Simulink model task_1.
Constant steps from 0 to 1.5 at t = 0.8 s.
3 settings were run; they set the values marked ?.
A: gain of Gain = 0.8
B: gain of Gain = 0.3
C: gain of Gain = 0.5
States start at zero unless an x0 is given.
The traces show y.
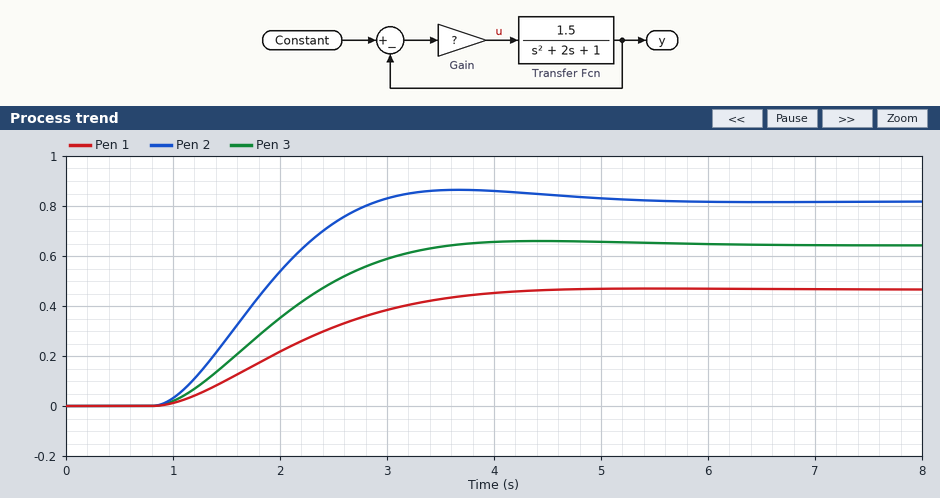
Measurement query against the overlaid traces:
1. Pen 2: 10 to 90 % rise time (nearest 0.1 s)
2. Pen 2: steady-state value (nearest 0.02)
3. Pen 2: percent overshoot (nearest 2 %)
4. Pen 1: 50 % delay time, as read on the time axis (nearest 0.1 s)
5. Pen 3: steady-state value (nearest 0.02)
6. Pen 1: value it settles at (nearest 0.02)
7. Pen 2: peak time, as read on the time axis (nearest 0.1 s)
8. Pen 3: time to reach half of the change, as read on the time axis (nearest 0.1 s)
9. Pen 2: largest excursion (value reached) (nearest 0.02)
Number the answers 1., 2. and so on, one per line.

1. 1.4 s
2. 0.82
3. 6 %
4. 2.1 s
5. 0.64
6. 0.46
7. 3.7 s
8. 1.9 s
9. 0.86
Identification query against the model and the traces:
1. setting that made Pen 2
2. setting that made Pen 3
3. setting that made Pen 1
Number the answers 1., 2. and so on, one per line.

1. A
2. C
3. B
